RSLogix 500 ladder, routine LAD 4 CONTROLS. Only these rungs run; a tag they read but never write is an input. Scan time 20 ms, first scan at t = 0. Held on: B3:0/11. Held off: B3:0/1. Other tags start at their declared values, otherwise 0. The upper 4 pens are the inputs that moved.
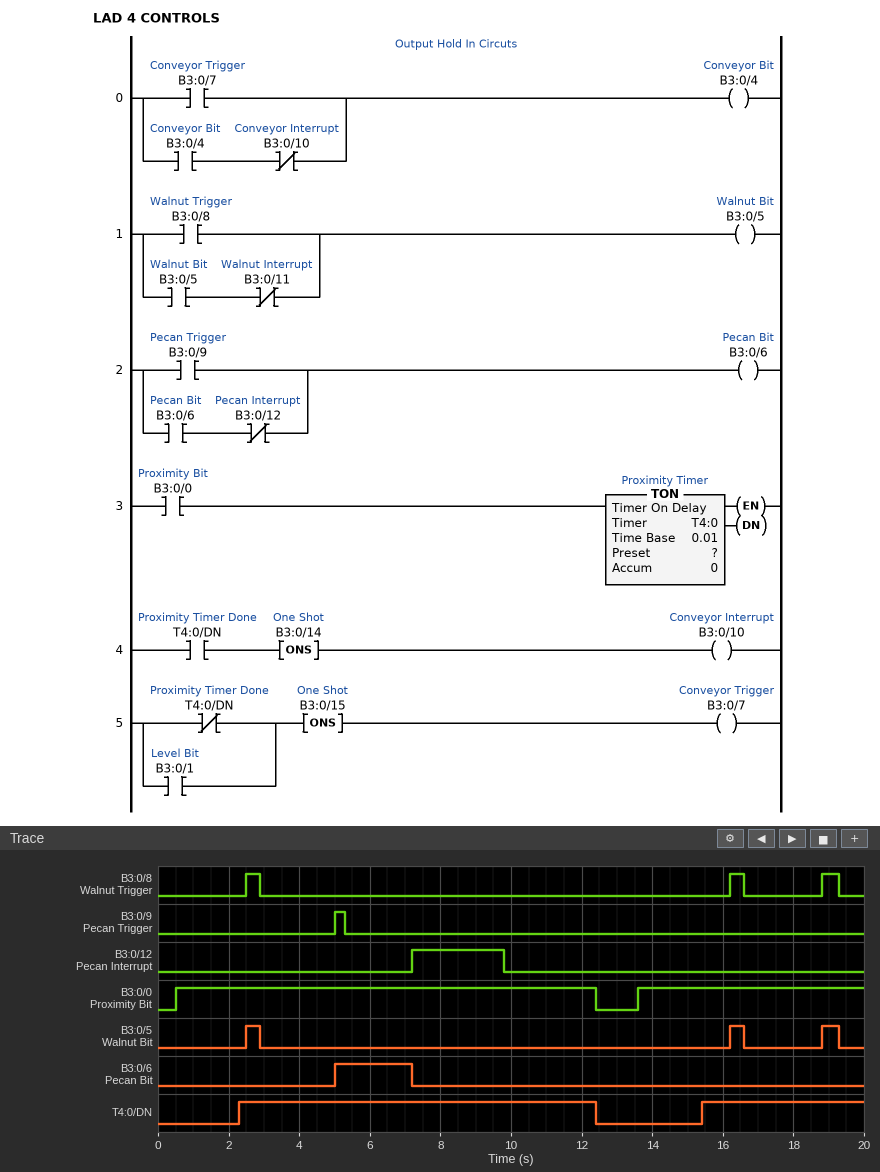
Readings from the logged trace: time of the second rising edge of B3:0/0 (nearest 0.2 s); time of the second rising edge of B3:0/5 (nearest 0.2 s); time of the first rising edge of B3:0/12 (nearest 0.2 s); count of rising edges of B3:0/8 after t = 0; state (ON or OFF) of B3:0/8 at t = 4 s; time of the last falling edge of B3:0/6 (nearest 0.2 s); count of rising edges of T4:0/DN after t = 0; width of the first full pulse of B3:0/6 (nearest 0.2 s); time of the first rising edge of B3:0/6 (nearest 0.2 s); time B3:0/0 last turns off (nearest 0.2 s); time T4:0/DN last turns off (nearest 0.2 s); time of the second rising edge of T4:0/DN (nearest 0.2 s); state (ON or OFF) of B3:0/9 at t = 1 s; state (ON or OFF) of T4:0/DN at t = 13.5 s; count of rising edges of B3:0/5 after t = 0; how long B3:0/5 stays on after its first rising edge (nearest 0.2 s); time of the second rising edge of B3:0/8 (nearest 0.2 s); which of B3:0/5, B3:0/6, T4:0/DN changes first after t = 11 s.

13.6 s
16.2 s
7.2 s
3
OFF
7.2 s
2
2.2 s
5.0 s
12.4 s
12.4 s
15.4 s
OFF
OFF
3
0.4 s
16.2 s
T4:0/DN
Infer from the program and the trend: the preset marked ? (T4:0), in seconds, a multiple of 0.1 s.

1.8 s
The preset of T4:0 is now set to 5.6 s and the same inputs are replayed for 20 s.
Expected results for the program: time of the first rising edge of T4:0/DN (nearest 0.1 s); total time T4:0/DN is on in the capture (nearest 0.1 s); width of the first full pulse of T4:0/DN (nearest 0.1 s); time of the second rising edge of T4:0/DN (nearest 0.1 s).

6.1 s
7.1 s
6.3 s
19.2 s
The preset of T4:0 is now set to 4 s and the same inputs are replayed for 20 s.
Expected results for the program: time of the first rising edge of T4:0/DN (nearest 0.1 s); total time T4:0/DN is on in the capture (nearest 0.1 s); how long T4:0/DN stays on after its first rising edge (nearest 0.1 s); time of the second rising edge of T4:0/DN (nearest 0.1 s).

4.5 s
10.3 s
7.9 s
17.6 s
